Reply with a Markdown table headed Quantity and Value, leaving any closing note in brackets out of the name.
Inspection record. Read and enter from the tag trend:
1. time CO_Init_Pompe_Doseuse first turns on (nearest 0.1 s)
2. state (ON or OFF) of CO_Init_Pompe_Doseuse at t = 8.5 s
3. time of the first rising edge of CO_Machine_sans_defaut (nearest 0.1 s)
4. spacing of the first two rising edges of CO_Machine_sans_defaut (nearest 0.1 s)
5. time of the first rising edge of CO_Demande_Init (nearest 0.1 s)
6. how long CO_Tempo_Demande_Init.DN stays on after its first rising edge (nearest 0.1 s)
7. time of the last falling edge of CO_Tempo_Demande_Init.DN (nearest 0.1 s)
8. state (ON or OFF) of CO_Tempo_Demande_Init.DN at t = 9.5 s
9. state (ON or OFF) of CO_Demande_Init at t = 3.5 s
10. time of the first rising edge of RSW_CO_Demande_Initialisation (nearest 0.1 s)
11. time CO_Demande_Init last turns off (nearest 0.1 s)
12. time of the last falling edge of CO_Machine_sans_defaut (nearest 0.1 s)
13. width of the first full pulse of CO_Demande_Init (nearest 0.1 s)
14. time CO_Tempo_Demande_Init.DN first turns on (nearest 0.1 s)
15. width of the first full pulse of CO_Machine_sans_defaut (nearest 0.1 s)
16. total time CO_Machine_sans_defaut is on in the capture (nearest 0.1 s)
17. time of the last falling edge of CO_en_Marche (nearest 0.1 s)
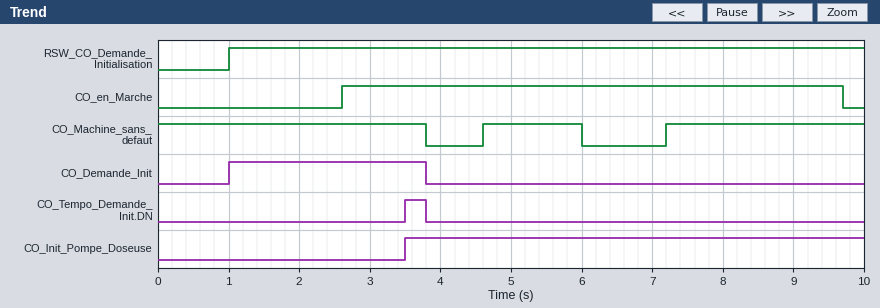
| Quantity | Value |
|---|---|
| time CO_Init_Pompe_Doseuse first turns on | 3.5 s |
| state (ON or OFF) of CO_Init_Pompe_Doseuse at t = 8.5 s | ON |
| time of the first rising edge of CO_Machine_sans_defaut | 4.6 s |
| spacing of the first two rising edges of CO_Machine_sans_defaut | 2.6 s |
| time of the first rising edge of CO_Demande_Init | 1.0 s |
| how long CO_Tempo_Demande_Init.DN stays on after its first rising edge | 0.3 s |
| time of the last falling edge of CO_Tempo_Demande_Init.DN | 3.8 s |
| state (ON or OFF) of CO_Tempo_Demande_Init.DN at t = 9.5 s | OFF |
| state (ON or OFF) of CO_Demande_Init at t = 3.5 s | ON |
| time of the first rising edge of RSW_CO_Demande_Initialisation | 1.0 s |
| time CO_Demande_Init last turns off | 3.8 s |
| time of the last falling edge of CO_Machine_sans_defaut | 6.0 s |
| width of the first full pulse of CO_Demande_Init | 2.8 s |
| time CO_Tempo_Demande_Init.DN first turns on | 3.5 s |
| width of the first full pulse of CO_Machine_sans_defaut | 1.4 s |
| total time CO_Machine_sans_defaut is on in the capture | 8.0 s |
| time of the last falling edge of CO_en_Marche | 9.7 s |
